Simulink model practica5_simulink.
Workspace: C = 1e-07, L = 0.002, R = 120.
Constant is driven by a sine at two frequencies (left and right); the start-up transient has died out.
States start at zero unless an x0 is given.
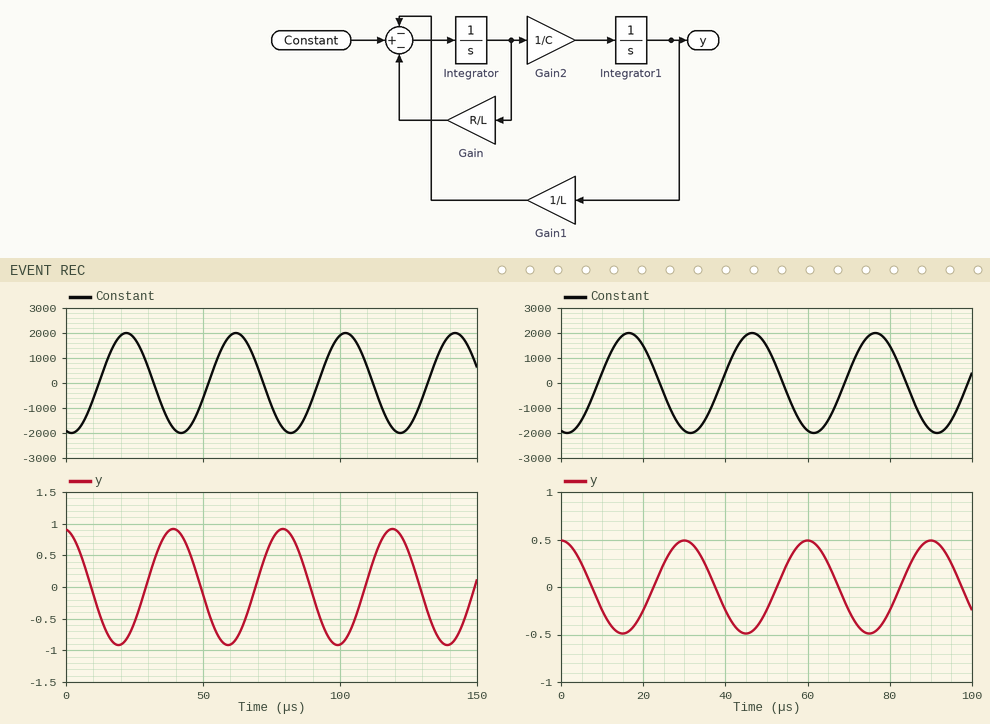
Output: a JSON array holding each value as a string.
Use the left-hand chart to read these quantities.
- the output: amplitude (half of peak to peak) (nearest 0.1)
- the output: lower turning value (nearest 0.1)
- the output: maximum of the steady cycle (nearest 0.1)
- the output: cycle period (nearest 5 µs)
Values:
["0.9", "-0.9", "0.9", "40 µs"]
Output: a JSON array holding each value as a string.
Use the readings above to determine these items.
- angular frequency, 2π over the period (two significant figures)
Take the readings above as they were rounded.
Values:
["0.16 rad/µs"]
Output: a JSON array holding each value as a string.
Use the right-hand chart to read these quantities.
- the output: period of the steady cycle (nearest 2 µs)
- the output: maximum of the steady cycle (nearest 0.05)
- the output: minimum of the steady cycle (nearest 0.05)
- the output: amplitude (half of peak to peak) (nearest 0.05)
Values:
["30 µs", "0.50", "-0.50", "0.50"]
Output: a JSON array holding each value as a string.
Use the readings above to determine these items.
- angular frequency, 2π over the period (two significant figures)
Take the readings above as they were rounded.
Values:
["0.21 rad/µs"]
